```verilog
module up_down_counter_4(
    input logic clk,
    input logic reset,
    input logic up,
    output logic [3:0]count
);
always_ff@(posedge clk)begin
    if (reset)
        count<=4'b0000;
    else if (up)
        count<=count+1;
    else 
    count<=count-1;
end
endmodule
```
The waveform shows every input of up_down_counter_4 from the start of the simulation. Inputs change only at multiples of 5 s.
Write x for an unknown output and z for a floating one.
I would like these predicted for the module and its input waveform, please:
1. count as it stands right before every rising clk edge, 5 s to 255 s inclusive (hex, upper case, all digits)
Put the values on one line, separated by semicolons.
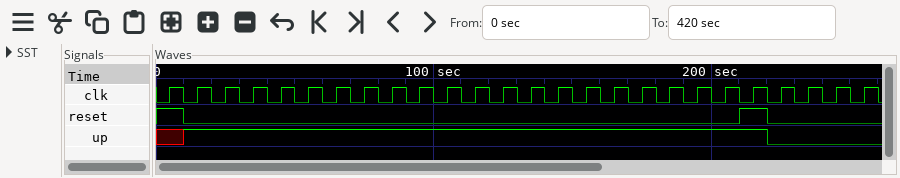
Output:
x, 0, 1, 2, 3, 4, 5, 6, 7, 8, 9, A, B, C, D, E, F, 0, 1, 2, 3, 4, 0, F, E, D
